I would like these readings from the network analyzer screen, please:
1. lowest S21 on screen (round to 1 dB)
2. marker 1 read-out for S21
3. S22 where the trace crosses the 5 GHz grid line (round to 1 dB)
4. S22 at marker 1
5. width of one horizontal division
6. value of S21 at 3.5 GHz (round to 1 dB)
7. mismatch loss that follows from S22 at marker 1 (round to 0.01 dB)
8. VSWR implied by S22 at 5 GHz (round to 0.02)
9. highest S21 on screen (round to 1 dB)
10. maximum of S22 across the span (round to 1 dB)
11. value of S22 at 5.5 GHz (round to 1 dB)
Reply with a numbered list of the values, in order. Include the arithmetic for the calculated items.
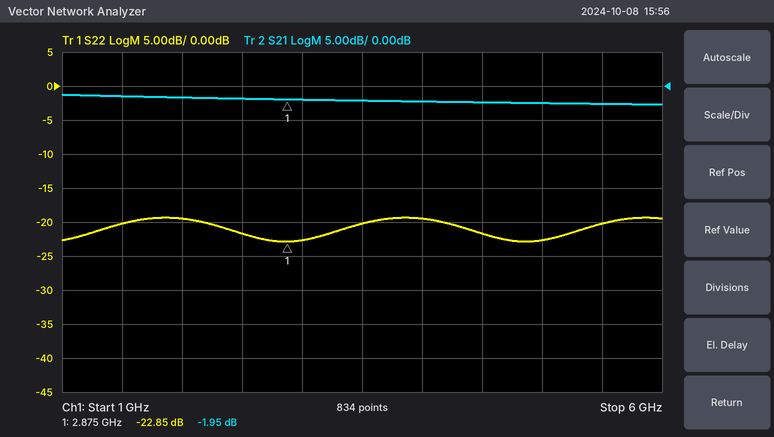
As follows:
1. -3 dB
2. -1.95 dB
3. -23 dB
4. -22.85 dB
5. 500 MHz
6. -2 dB
7. −10 log10(1 − 10^(-22.85/10)) ≈ 0.02 dB
8. |Γ| = 10^(-23/20) = 0.0708; VSWR = (1 + 0.0708)/(1 − 0.0708) ≈ 1.15, so 1.16 to the nearest 0.02
9. -1 dB
10. -19 dB
11. -20 dB
